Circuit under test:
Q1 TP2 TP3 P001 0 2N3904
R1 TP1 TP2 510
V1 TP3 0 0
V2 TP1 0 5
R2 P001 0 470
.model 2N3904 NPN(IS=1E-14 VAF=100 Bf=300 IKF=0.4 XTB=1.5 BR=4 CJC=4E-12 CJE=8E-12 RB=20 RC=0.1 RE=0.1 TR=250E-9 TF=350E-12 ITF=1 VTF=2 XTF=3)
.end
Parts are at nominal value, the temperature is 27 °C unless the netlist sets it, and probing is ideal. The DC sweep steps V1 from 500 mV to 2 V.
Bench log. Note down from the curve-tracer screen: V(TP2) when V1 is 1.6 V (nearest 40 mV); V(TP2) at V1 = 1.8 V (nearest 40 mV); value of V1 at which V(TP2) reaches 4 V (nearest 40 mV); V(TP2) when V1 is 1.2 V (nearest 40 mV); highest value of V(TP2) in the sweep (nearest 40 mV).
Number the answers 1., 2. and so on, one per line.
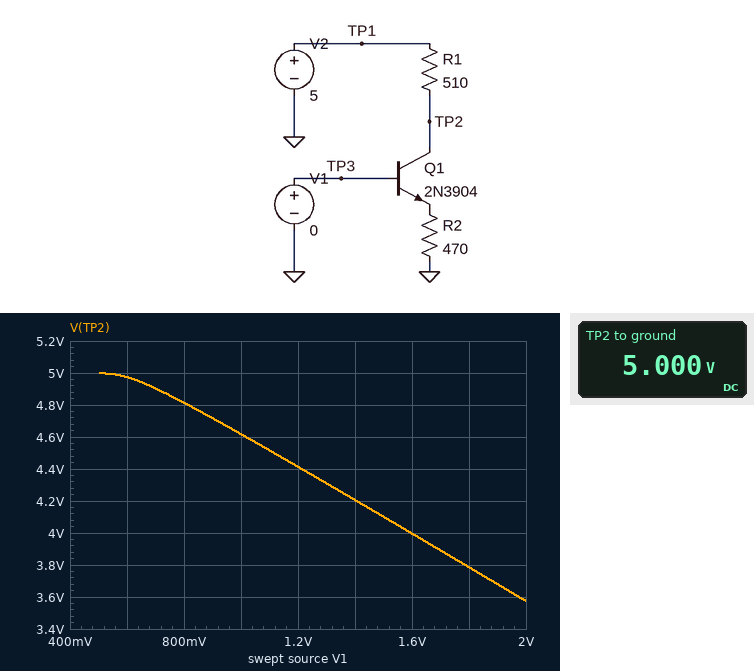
1. 4.00 V
2. 3.80 V
3. 1.60 V
4. 4.40 V
5. 5.00 V
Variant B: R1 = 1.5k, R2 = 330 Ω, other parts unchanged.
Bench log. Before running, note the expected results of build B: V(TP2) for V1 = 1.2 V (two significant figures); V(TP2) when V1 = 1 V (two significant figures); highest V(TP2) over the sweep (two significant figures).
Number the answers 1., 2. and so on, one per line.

1. 2.6 V
2. 3.4 V
3. 5.0 V
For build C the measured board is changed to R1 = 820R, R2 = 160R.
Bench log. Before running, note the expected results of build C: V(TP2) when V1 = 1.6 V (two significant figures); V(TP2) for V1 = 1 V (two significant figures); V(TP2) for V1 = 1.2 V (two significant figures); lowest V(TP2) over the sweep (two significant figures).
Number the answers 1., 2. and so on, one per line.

1. 920 mV
2. 3.3 V
3. 2.4 V
4. 890 mV
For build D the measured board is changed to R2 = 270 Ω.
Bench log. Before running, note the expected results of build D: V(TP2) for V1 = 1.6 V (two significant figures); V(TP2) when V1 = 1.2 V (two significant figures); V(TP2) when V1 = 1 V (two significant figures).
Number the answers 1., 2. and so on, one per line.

1. 3.3 V
2. 4.0 V
3. 4.4 V
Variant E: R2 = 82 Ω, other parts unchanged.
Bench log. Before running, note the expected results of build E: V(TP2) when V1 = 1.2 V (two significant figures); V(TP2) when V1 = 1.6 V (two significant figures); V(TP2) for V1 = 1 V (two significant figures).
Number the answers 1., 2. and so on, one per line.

1. 1.9 V
2. 850 mV
3. 3.1 V
